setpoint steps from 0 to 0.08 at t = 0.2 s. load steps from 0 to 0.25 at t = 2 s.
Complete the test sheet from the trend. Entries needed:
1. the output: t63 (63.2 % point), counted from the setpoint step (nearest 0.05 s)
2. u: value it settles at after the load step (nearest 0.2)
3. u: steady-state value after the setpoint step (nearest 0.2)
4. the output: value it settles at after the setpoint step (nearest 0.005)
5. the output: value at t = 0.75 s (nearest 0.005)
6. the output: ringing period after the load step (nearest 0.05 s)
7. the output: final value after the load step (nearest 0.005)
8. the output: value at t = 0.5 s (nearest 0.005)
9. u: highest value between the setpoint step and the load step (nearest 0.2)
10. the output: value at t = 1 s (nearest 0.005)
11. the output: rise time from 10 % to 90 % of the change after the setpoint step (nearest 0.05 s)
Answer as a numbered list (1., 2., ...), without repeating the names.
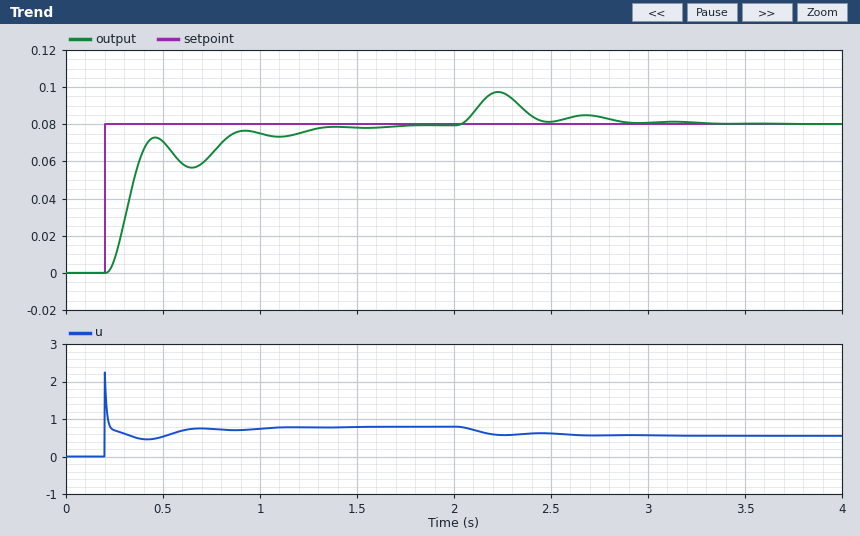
1. 0.15 s
2. 0.6
3. 0.8
4. 0.080
5. 0.065
6. 0.45 s
7. 0.080
8. 0.070
9. 2.2
10. 0.075
11. 0.20 s
